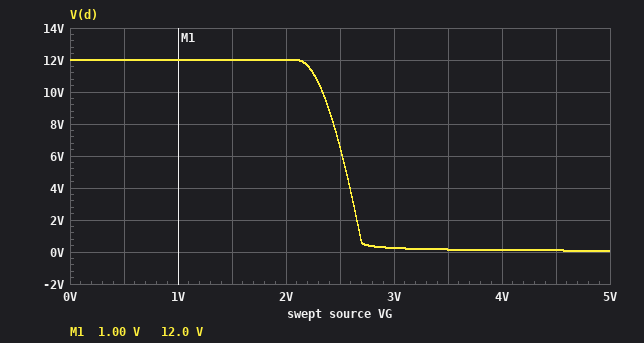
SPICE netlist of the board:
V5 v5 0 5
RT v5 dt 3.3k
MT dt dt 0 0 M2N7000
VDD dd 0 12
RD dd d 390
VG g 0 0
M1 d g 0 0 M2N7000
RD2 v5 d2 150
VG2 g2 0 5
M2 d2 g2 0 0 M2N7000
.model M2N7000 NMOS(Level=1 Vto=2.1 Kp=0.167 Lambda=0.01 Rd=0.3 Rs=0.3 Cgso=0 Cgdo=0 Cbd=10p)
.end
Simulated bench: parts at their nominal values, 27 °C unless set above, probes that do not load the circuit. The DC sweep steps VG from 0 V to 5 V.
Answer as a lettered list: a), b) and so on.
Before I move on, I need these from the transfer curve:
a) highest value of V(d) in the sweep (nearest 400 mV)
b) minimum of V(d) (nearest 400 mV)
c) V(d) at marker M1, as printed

a) 12.0 V
b) 0 V
c) 12.0 V
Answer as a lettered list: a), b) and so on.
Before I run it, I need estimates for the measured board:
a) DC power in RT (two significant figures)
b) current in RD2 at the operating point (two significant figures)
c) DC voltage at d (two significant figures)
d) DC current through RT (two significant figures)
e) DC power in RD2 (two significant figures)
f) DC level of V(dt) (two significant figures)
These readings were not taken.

a) 2.4 mW
b) 33 mA
c) 12 V
d) 850 µA
e) 160 mW
f) 2.2 V
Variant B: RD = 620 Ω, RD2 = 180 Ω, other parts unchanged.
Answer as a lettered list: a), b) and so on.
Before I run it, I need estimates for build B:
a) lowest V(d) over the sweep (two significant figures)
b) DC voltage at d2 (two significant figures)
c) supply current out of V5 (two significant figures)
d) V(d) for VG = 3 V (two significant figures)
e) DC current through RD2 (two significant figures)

a) 52 mV
b) 74 mV
c) 28 mA
d) 150 mV
e) 27 mA
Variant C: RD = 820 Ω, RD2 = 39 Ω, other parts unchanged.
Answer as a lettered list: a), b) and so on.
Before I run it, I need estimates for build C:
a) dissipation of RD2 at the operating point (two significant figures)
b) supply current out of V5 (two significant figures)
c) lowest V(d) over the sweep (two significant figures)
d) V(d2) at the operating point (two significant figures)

a) 560 mW
b) 120 mA
c) 39 mV
d) 330 mV
